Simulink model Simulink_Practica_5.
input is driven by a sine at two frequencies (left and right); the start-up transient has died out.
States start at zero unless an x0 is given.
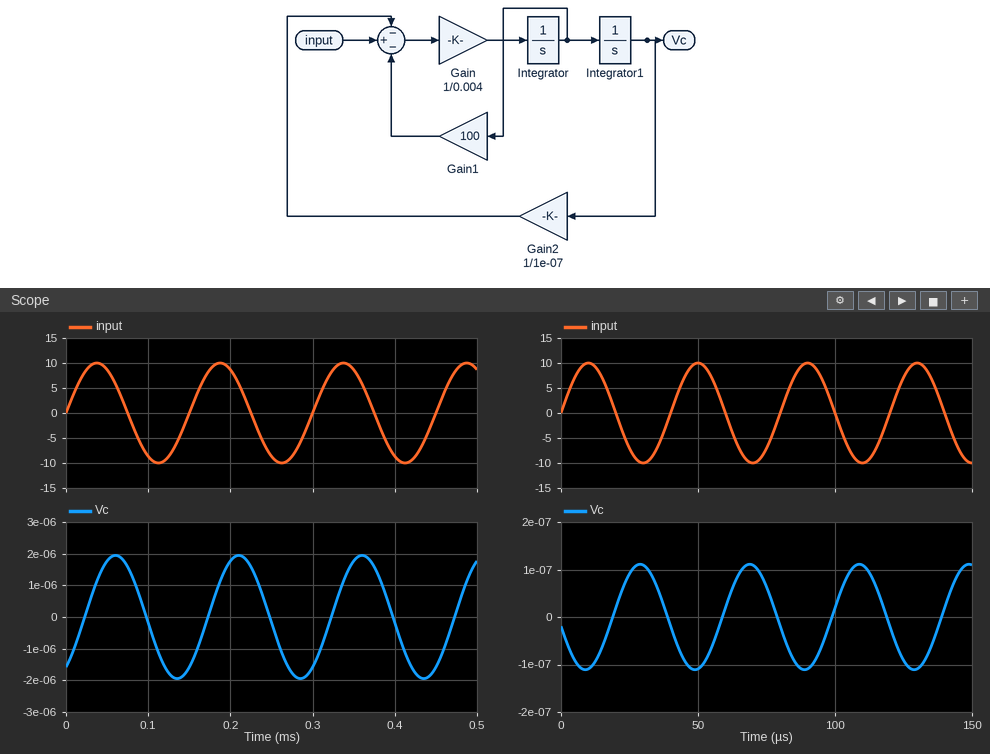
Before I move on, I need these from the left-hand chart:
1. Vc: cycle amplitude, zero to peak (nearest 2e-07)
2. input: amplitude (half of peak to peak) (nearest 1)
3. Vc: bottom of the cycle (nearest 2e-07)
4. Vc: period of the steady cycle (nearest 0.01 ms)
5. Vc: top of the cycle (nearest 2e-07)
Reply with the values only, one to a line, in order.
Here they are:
0.0000020
10
-0.0000020
0.15 ms
0.0000020
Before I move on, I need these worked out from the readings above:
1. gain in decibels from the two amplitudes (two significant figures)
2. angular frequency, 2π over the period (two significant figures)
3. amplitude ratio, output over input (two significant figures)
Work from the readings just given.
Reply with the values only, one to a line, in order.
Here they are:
-130 dB
42 rad/ms
0.00000020
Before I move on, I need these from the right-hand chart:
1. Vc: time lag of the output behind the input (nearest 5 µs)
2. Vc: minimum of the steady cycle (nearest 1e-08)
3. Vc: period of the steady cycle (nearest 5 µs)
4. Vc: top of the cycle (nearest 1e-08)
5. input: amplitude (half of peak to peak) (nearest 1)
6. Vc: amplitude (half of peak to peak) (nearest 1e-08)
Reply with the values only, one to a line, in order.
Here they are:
20 µs
-0.00000011
40 µs
0.00000011
10
0.00000011
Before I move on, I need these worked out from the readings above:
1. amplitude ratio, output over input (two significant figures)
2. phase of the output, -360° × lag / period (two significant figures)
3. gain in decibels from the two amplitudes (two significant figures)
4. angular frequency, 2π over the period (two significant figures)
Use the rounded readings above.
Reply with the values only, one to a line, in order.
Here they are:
0.000000011
-180°
-160 dB
0.16 rad/µs
